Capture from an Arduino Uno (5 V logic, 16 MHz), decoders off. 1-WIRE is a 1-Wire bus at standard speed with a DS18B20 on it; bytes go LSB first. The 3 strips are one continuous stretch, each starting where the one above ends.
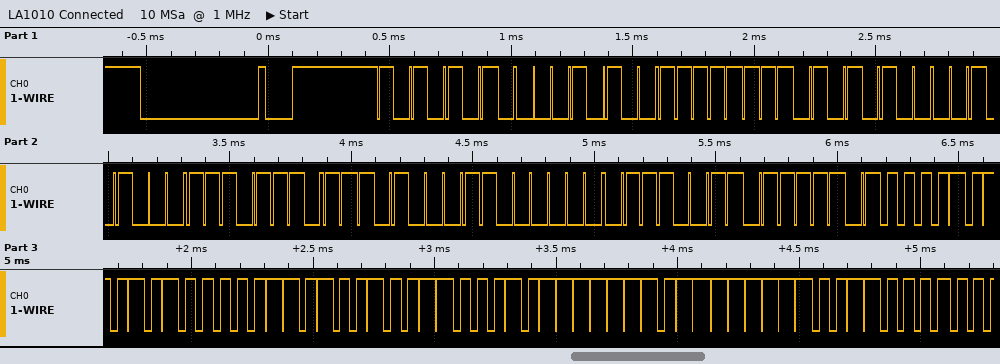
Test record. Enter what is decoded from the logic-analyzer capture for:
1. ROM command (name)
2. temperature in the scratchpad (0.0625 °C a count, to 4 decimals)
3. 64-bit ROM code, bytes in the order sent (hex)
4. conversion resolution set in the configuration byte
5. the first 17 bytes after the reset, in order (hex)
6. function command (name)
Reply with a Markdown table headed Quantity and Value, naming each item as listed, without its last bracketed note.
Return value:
| Quantity | Value |
|---|---|
| ROM command | Match ROM |
| temperature in the scratchpad | 85.0000 °C |
| 64-bit ROM code, bytes in the order sent | 28 FF 2A 14 77 17 03 CE |
| conversion resolution set in the configuration byte | 12 bits |
| the first 17 bytes after the reset, in order | 55 28 FF 2A 14 77 17 03 CE BE 50 05 4B 46 7F FF 0C |
| function command | Read Scratchpad |
